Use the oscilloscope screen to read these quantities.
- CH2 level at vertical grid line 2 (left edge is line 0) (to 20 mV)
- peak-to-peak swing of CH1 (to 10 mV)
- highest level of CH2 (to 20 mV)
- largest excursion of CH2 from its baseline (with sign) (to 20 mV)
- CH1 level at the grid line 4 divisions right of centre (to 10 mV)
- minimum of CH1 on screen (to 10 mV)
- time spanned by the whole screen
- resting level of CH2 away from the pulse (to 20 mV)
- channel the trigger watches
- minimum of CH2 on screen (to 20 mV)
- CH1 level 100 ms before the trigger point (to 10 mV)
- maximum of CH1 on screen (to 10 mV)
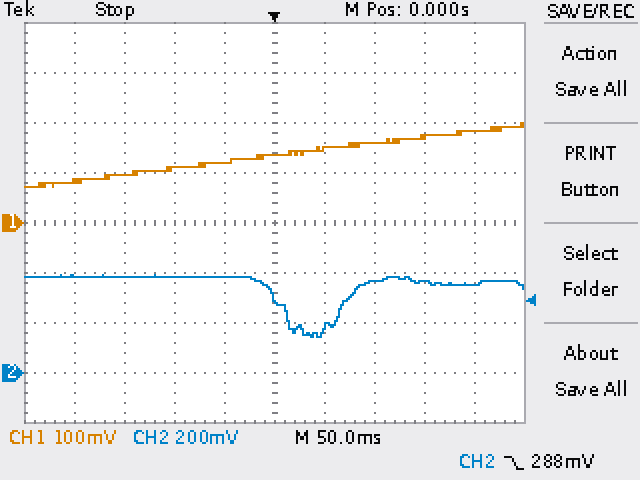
380 mV
130 mV
400 mV
-240 mV
180 mV
70 mV
500 ms
380 mV
CH2
140 mV
110 mV
200 mV
